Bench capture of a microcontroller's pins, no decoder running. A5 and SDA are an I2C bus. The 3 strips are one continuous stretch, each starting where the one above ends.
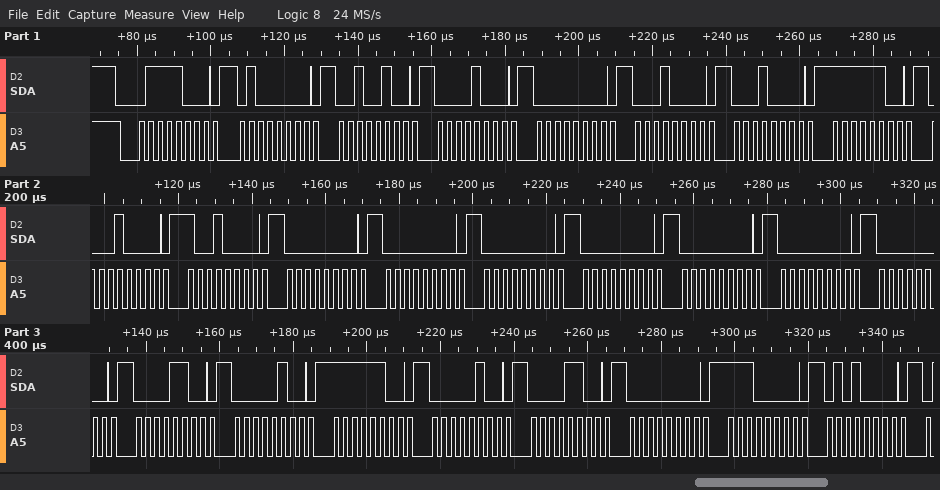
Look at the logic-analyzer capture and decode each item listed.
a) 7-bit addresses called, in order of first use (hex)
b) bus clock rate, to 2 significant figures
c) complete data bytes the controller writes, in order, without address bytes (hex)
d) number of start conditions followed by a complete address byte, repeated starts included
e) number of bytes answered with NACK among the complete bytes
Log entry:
0x3C
400 kHz
40 24 08 00 10 10 FC 10 90 00 00 00 00 00 00 00 0C 04 FC 04 0C 00 E0 50
1
0
